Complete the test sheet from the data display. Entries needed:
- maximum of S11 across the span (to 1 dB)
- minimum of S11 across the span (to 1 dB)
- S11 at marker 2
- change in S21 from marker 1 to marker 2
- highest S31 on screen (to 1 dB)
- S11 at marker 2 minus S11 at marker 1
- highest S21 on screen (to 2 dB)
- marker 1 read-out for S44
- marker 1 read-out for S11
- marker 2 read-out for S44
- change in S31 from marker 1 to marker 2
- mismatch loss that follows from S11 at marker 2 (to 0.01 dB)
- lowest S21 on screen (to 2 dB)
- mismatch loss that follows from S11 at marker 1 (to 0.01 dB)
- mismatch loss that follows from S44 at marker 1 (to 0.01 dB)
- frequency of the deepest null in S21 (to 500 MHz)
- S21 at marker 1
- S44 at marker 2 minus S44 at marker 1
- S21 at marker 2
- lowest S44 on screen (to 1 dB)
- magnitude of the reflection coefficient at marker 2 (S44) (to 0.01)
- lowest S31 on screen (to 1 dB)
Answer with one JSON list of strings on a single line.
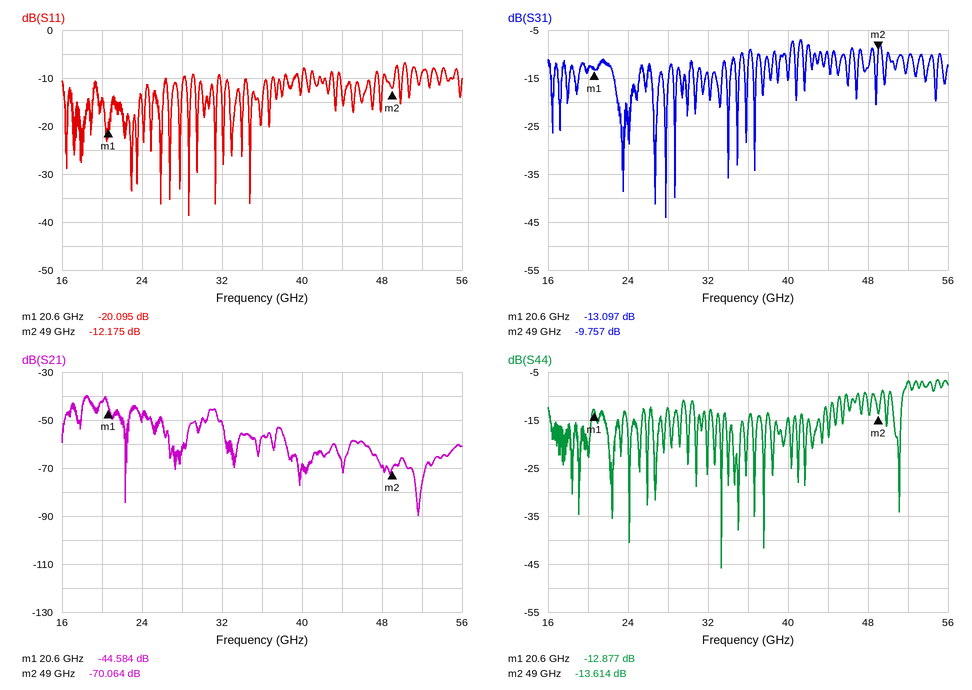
["-7 dB", "-39 dB", "-12.175 dB", "-25.480 dB", "-7 dB", "7.920 dB", "-40 dB", "-12.877 dB", "-20.095 dB", "-13.614 dB", "3.340 dB", "0.27 dB", "-90 dB", "0.04 dB", "0.23 dB", "51.5 GHz", "-44.584 dB", "-0.737 dB", "-70.064 dB", "-46 dB", "0.21", "-44 dB"]
